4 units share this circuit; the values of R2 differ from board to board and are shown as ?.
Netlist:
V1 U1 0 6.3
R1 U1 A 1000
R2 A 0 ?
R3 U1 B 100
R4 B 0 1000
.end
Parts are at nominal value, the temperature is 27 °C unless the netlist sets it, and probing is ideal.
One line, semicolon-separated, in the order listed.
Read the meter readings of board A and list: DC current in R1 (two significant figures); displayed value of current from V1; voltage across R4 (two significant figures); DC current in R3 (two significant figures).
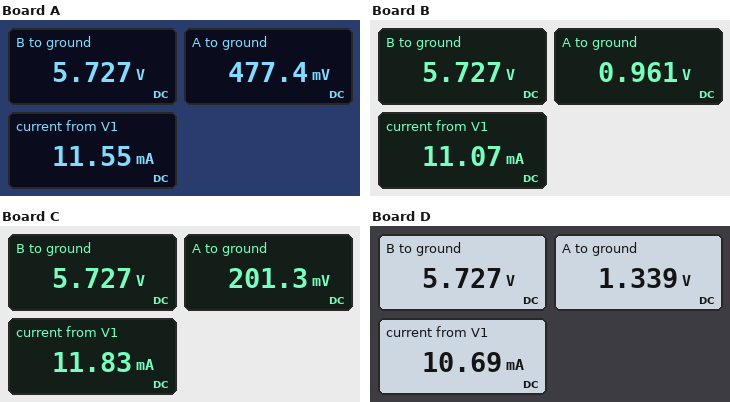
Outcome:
5.8 mA; 11.55 mA; 5.7 V; 5.7 mA
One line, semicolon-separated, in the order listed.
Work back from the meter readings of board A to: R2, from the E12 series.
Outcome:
82 Ω
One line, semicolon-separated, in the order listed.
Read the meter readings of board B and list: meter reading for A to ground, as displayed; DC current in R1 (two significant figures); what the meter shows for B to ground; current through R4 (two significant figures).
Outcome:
0.961 V; 5.3 mA; 5.727 V; 5.7 mA
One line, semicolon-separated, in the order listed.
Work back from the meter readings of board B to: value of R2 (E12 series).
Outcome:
180 Ω
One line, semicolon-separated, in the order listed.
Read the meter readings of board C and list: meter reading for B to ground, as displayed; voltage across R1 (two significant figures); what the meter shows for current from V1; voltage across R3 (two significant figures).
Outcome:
5.727 V; 6.1 V; 11.83 mA; 570 mV
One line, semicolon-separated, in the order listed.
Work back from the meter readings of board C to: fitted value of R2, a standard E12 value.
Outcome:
33 Ω
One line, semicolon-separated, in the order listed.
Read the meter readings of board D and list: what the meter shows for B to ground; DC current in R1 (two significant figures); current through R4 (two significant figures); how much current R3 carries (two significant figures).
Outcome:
5.727 V; 5.0 mA; 5.7 mA; 5.7 mA
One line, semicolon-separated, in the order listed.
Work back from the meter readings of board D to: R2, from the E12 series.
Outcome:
270 Ω
